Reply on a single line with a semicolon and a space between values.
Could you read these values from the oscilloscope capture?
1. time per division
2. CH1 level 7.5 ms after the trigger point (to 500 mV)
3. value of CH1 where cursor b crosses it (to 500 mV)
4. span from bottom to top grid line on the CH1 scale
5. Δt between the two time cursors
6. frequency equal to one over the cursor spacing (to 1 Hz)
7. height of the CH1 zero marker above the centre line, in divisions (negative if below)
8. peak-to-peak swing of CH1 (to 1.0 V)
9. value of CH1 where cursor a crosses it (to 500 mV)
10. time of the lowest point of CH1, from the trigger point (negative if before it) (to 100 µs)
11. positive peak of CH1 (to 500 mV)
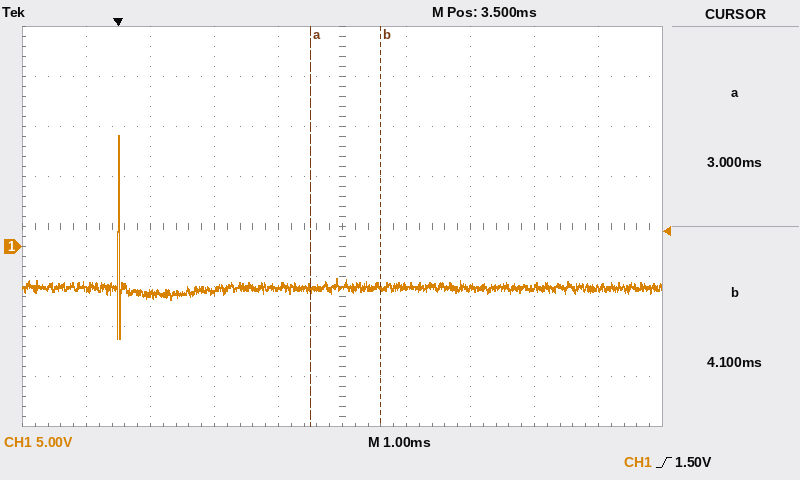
1 ms; -4.0 V; -4.0 V; 40 V; 1.1 ms; 909 Hz; -0.4 div; 20.0 V; -4.0 V; 0.0 ms; 11.0 V
